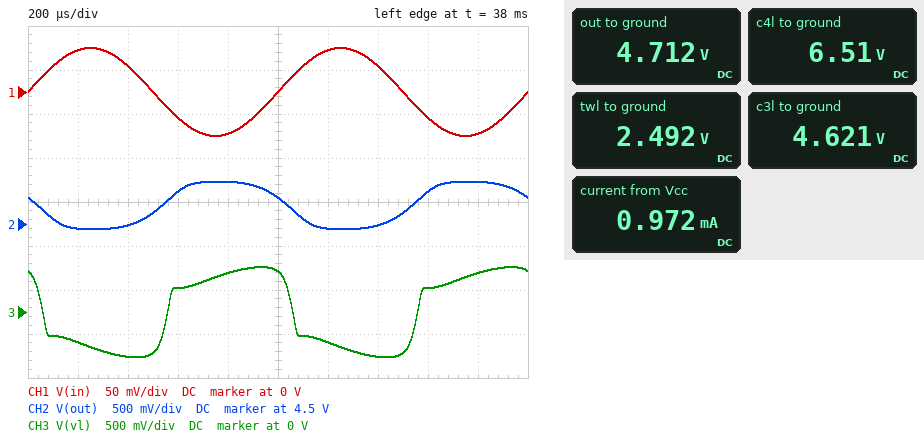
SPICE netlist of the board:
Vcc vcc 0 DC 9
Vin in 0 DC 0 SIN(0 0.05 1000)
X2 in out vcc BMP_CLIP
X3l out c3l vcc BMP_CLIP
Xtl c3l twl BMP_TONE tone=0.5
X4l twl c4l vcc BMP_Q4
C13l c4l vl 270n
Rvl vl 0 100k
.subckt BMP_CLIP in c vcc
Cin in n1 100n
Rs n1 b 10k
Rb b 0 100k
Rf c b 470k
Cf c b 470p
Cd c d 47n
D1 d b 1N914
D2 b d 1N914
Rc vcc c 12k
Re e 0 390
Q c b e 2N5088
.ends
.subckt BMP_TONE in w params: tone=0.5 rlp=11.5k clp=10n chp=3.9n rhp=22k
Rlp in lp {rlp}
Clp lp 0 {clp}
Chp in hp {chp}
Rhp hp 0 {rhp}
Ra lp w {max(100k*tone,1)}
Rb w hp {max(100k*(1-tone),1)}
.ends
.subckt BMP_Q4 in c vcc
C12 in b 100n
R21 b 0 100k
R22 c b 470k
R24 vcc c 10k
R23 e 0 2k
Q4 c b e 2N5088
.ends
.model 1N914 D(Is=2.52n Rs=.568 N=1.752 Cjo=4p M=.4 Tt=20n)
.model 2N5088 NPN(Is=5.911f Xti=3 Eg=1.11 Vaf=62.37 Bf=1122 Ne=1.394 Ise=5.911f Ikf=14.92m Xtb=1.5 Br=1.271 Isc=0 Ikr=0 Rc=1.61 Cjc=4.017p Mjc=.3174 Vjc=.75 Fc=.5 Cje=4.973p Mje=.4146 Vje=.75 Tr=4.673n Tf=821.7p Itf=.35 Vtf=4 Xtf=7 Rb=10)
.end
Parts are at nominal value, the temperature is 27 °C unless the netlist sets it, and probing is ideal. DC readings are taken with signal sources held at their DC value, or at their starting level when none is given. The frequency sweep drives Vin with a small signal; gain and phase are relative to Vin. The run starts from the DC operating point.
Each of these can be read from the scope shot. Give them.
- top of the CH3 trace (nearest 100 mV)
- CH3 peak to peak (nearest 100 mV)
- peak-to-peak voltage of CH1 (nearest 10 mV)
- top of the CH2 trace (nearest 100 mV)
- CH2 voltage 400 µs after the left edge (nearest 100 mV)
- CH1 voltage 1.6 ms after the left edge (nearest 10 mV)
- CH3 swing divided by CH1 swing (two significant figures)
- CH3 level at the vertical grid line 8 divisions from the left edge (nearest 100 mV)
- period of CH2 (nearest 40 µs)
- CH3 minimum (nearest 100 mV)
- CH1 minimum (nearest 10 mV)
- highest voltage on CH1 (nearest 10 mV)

500 mV
1.0 V
100 mV
5.0 V
4.5 V
-30 mV
10
300 mV
1.00 ms
-500 mV
-50 mV
50 mV
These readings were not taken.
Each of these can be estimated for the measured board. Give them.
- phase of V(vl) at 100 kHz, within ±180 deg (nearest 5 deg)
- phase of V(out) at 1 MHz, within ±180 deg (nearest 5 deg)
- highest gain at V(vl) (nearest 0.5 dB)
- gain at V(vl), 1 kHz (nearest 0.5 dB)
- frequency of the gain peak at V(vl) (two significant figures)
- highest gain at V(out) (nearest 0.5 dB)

-20 deg
35 deg
44.5 dB
40.0 dB
220 Hz
20.5 dB
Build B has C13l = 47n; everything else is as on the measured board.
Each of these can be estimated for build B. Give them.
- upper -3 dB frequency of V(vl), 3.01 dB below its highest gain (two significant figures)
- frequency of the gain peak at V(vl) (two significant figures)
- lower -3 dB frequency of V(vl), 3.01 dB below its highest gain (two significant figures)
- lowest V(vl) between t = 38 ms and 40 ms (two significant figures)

800 Hz
230 Hz
77 Hz
-510 mV
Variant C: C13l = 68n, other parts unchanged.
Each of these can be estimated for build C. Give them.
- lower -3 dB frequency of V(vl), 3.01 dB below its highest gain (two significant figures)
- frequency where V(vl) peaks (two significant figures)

74 Hz
230 Hz
